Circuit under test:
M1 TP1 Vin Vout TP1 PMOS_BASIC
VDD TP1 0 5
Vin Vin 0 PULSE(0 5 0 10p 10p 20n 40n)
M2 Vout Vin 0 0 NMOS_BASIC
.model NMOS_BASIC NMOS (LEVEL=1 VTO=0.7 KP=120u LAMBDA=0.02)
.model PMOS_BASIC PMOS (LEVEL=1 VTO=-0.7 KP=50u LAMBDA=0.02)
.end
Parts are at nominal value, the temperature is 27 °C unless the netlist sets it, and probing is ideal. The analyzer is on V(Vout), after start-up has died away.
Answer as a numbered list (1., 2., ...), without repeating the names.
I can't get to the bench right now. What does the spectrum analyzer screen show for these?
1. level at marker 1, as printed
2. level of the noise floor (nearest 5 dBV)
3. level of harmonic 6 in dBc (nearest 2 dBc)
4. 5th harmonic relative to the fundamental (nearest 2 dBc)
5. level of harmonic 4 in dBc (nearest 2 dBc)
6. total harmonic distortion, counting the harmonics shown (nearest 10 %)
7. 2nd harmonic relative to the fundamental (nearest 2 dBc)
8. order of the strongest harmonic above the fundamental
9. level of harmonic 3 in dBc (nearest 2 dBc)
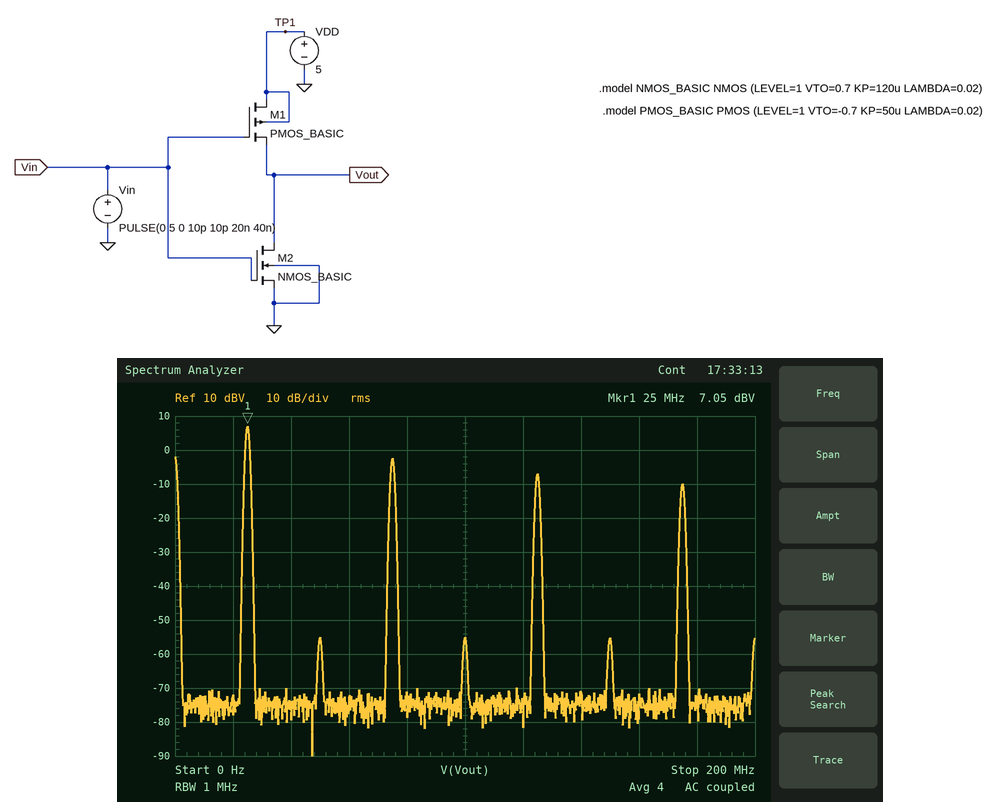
1. 7.05 dBV
2. -75 dBV
3. -62 dBc
4. -14 dBc
5. -62 dBc
6. 40 %
7. -62 dBc
8. 3
9. -10 dBc
